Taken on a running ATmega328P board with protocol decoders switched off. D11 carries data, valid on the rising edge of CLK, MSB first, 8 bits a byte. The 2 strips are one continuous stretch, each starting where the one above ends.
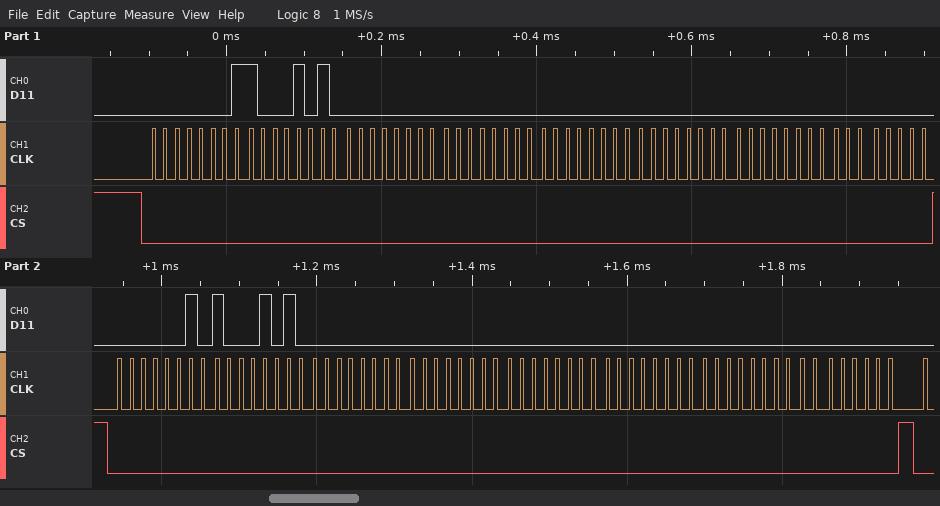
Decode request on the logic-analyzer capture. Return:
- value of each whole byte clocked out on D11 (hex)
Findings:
0x01 0x8A 0x00 0x00 0x00 0x00 0x00 0x00 0x02 0x8A 0x00 0x00 0x00 0x00 0x00 0x00
